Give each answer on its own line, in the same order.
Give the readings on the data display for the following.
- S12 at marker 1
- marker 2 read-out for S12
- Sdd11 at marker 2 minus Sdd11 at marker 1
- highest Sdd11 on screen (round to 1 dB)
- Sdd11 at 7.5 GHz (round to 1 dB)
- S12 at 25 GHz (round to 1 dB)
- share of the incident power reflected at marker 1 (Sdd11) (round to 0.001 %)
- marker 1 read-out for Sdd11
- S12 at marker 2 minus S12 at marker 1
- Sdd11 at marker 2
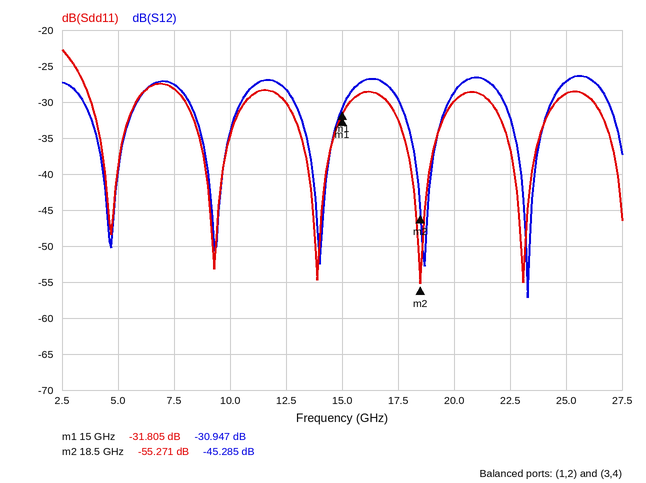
-30.947 dB
-45.285 dB
-23.466 dB
-23 dB
-28 dB
-27 dB
0.066 %
-31.805 dB
-14.338 dB
-55.271 dB
